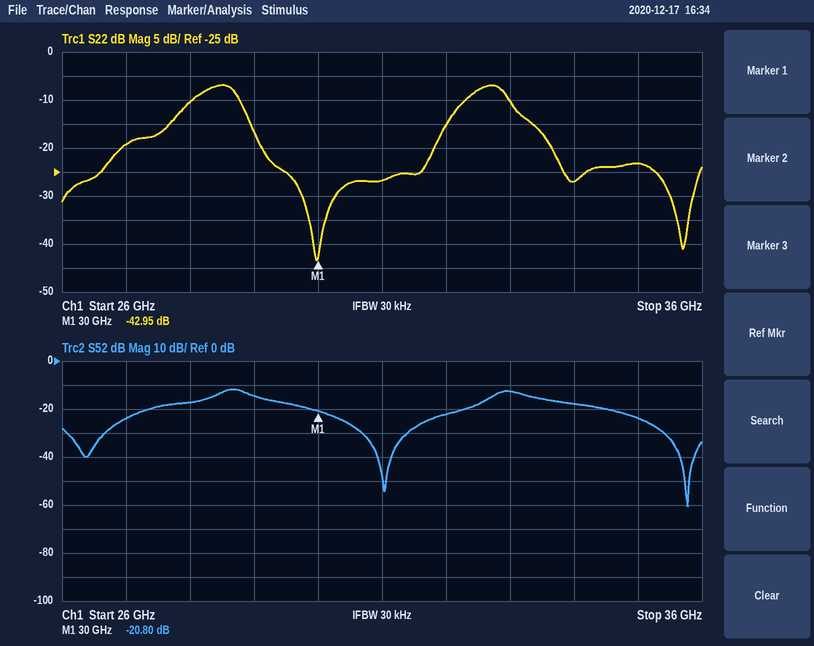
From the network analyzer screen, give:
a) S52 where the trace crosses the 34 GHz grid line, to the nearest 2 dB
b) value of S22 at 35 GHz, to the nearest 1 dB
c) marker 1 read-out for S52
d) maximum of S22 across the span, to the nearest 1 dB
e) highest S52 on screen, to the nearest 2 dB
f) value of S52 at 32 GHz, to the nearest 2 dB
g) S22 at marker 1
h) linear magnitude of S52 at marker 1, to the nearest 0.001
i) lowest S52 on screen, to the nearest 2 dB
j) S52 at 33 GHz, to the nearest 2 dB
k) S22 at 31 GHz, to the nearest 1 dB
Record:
-18 dB
-23 dB
-20.80 dB
-7 dB
-12 dB
-22 dB
-42.95 dB
0.091
-60 dB
-12 dB
-27 dB
